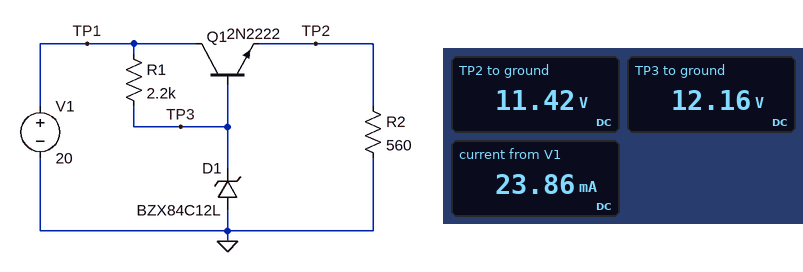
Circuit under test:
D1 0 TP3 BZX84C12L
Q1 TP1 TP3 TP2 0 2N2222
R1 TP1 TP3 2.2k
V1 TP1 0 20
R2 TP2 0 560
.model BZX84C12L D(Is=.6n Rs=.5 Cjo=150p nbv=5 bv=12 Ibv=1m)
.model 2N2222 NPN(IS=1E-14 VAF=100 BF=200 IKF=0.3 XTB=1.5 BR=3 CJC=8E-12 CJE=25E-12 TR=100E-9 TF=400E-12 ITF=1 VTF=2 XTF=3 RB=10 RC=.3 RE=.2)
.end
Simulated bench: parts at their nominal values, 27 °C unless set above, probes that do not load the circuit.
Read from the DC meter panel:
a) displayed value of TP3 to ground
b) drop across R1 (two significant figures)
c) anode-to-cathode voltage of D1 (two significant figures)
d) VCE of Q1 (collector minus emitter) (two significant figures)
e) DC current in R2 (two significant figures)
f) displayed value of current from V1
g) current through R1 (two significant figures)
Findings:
12.16 V
7.8 V
-12 V
8.6 V
20 mA
23.86 mA
3.6 mA
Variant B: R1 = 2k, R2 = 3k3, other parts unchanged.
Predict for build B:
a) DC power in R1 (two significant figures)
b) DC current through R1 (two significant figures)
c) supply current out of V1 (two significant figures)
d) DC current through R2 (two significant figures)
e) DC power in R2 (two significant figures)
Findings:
31 mW
3.9 mA
7.4 mA
3.5 mA
40 mW
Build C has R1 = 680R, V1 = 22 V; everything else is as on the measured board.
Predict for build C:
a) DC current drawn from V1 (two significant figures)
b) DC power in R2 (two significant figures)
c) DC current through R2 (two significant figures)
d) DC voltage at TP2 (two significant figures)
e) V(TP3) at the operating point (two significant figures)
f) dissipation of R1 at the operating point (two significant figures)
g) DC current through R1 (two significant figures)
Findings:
35 mA
240 mW
21 mA
12 V
12 V
140 mW
14 mA
